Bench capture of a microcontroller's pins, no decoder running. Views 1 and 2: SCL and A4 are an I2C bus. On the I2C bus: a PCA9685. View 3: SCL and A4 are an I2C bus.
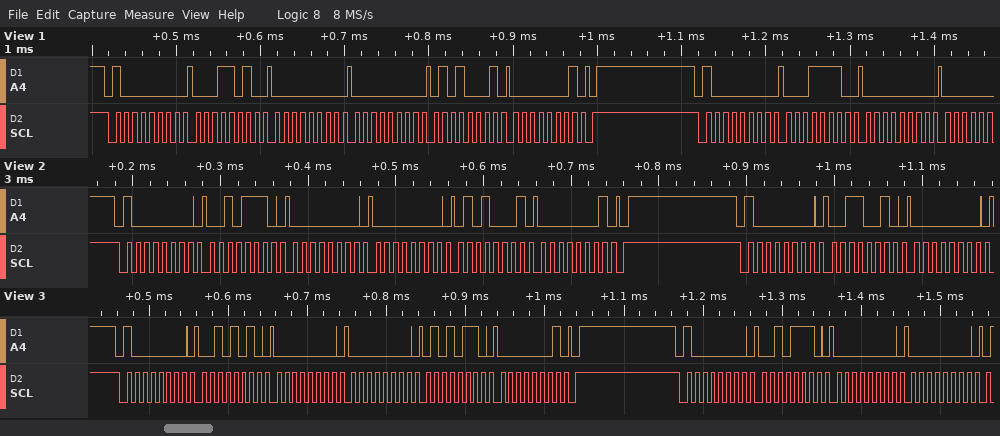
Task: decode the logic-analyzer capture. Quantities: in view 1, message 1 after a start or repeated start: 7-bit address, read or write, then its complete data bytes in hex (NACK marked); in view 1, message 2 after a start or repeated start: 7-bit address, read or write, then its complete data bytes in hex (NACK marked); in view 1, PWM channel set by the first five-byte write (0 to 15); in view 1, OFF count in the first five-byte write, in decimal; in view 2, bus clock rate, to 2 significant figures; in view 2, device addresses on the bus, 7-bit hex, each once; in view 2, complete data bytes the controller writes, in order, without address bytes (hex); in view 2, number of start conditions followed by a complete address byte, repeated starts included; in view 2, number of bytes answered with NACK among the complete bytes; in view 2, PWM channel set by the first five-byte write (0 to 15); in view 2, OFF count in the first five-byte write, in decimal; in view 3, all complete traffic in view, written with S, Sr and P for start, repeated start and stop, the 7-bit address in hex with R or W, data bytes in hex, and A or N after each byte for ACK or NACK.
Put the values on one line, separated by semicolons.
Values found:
0x40 write: 1A 00 00 51 01; 0x40 write: 1E 00; 5; 337; 100 kHz; 0x40; 2E 00 00 51 01 32 00; 2; 0; 10; 337; S 40W A 2A A 00 A 00 A 56 A 01 A P S 40W A 2E A 00 A 00 A
